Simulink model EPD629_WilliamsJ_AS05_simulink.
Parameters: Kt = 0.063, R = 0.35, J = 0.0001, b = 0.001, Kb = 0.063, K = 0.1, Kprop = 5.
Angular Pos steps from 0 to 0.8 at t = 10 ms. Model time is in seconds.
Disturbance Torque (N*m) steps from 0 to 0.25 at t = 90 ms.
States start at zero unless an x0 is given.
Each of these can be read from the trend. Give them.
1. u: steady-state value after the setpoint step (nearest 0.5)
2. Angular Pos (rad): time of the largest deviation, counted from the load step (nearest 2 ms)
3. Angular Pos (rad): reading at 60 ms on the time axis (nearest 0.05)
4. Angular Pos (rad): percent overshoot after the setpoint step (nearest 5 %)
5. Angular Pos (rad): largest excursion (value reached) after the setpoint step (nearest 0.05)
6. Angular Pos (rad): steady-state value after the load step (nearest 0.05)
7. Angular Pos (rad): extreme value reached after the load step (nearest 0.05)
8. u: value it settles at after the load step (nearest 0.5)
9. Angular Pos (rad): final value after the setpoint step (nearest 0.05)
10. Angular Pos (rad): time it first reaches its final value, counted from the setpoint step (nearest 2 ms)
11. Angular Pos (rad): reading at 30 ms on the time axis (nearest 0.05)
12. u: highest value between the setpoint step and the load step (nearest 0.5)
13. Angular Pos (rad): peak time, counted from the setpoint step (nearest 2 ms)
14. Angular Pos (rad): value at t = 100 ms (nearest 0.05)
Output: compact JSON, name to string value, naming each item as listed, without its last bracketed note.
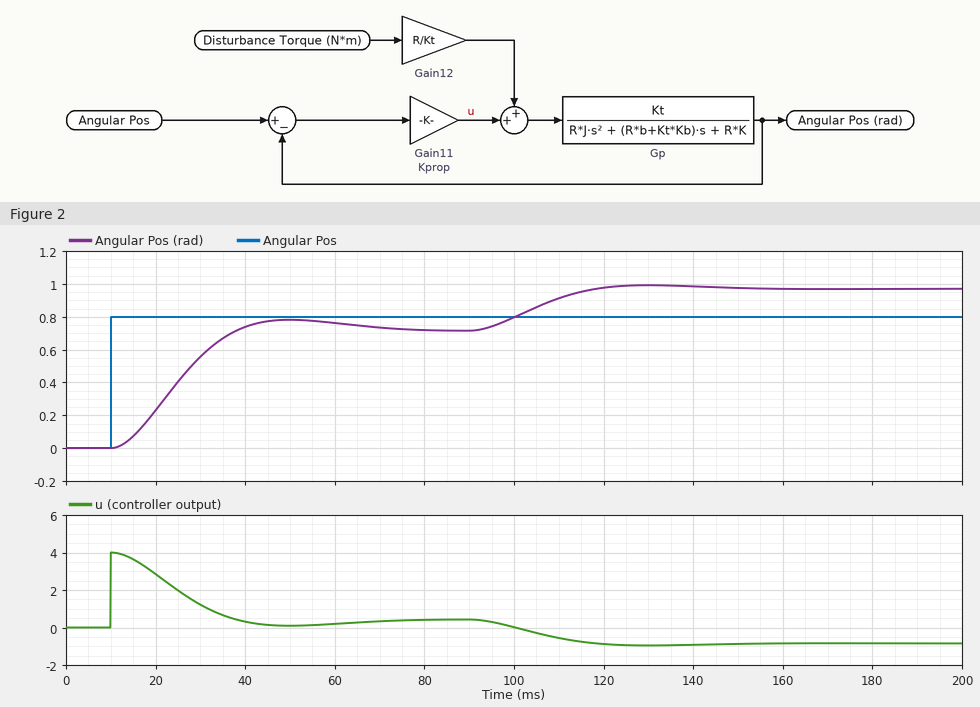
{"u: steady-state value after the setpoint step": "0.5", "Angular Pos (rad): time of the largest deviation, counted from the load step": "40 ms", "Angular Pos (rad): reading at 60 ms on the time axis": "0.75", "Angular Pos (rad): percent overshoot after the setpoint step": "10 %", "Angular Pos (rad): largest excursion (value reached) after the setpoint step": "0.80", "Angular Pos (rad): steady-state value after the load step": "0.95", "Angular Pos (rad): extreme value reached after the load step": "1.00", "u: value it settles at after the load step": "-1.0", "Angular Pos (rad): final value after the setpoint step": "0.70", "Angular Pos (rad): time it first reaches its final value, counted from the setpoint step": "28 ms", "Angular Pos (rad): reading at 30 ms on the time axis": "0.55", "u: highest value between the setpoint step and the load step": "4.0", "Angular Pos (rad): peak time, counted from the setpoint step": "40 ms", "Angular Pos (rad): value at t = 100 ms": "0.80"}
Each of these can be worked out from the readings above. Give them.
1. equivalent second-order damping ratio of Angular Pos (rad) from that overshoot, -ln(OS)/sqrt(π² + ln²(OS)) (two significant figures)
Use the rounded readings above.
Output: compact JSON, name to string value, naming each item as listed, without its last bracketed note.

{"equivalent second-order damping ratio of Angular Pos (rad) from that overshoot, -ln(OS)/sqrt(π² + ln²(OS))": "0.59"}
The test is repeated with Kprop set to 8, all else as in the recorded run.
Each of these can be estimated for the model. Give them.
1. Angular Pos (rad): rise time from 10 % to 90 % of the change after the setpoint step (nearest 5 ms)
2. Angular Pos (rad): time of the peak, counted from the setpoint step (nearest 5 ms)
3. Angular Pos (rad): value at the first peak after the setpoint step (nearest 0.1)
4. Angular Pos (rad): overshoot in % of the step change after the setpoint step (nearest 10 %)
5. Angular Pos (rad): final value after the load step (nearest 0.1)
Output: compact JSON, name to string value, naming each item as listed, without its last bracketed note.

{"Angular Pos (rad): rise time from 10 % to 90 % of the change after the setpoint step": "15 ms", "Angular Pos (rad): time of the peak, counted from the setpoint step": "30 ms", "Angular Pos (rad): value at the first peak after the setpoint step": "0.9", "Angular Pos (rad): overshoot in % of the step change after the setpoint step": "20 %", "Angular Pos (rad): final value after the load step": "0.9"}
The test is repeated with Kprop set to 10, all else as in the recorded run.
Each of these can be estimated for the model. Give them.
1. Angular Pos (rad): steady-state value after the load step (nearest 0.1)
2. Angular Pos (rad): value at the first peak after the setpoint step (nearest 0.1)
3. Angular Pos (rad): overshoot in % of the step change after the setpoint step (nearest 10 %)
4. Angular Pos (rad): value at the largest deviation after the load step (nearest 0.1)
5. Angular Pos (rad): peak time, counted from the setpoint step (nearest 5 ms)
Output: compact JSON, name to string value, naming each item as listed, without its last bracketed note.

{"Angular Pos (rad): steady-state value after the load step": "0.9", "Angular Pos (rad): value at the first peak after the setpoint step": "0.9", "Angular Pos (rad): overshoot in % of the step change after the setpoint step": "20 %", "Angular Pos (rad): value at the largest deviation after the load step": "0.9", "Angular Pos (rad): peak time, counted from the setpoint step": "25 ms"}
